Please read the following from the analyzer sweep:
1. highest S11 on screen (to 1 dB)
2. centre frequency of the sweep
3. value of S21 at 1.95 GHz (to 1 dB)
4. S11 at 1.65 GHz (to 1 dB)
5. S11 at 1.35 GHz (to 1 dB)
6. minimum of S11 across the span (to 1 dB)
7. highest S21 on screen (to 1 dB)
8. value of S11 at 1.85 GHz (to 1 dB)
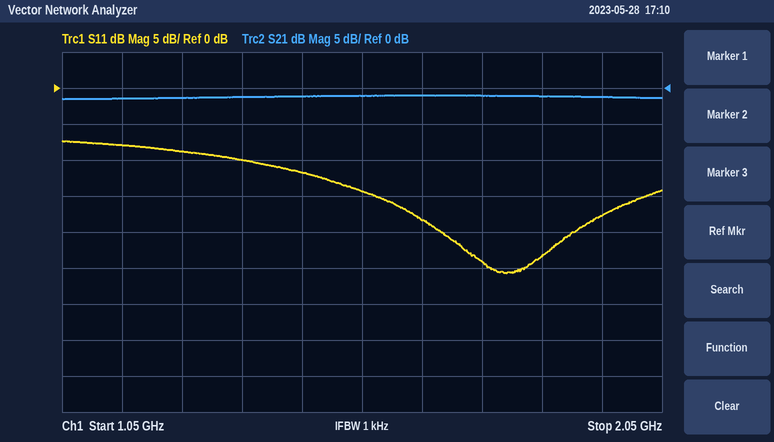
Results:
-7 dB
1.55 GHz
-1 dB
-18 dB
-10 dB
-26 dB
-1 dB
-23 dB
